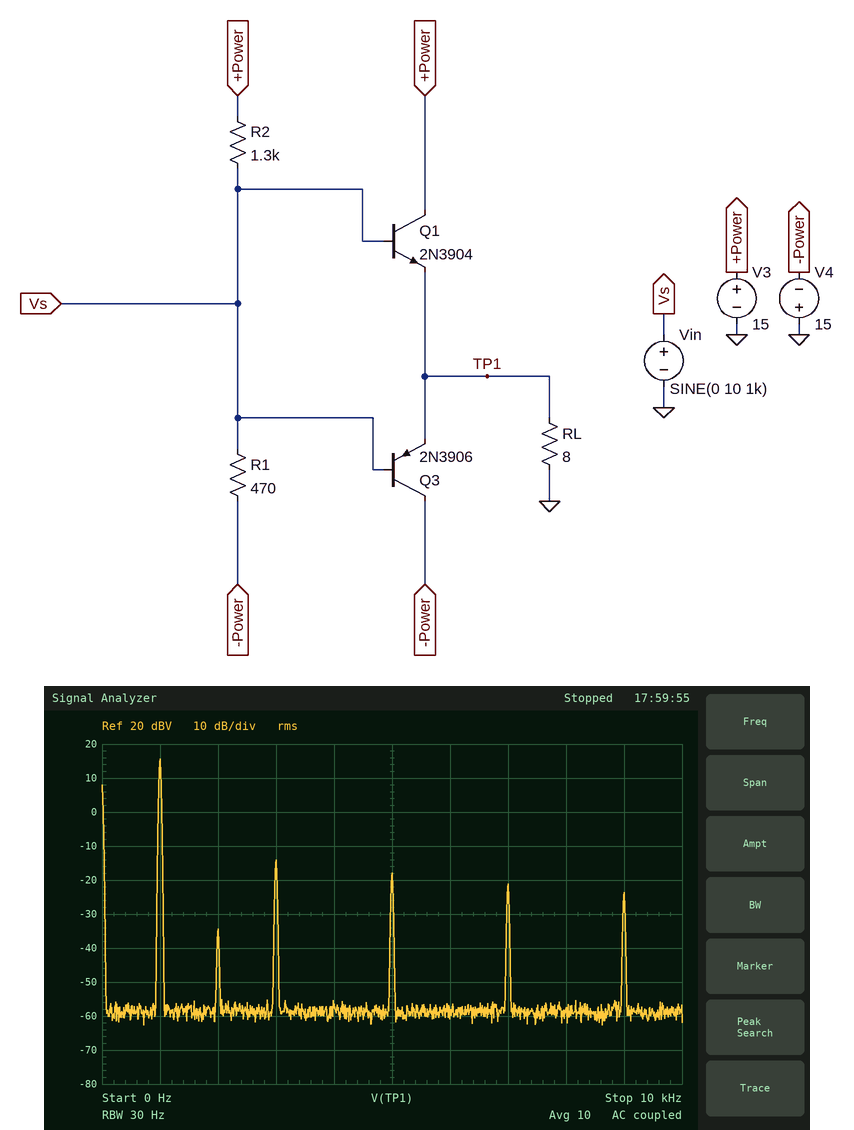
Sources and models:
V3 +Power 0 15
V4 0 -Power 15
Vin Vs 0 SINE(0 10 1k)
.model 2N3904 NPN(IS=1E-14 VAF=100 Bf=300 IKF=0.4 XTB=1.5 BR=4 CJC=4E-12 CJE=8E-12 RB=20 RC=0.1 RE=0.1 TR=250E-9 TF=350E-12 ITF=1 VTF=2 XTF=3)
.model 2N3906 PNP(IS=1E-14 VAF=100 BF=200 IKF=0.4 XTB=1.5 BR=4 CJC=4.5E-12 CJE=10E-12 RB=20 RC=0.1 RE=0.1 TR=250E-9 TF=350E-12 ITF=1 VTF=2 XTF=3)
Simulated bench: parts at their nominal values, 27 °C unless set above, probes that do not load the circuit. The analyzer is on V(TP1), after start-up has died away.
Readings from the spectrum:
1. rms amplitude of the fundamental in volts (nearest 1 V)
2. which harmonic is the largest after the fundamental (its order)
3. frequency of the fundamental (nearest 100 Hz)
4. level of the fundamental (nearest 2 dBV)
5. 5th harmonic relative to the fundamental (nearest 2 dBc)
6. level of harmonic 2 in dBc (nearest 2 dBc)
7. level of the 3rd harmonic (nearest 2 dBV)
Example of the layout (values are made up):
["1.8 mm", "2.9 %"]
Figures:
["6 V", "3", "1.0 kHz", "16 dBV", "-34 dBc", "-50 dBc", "-14 dBV"]
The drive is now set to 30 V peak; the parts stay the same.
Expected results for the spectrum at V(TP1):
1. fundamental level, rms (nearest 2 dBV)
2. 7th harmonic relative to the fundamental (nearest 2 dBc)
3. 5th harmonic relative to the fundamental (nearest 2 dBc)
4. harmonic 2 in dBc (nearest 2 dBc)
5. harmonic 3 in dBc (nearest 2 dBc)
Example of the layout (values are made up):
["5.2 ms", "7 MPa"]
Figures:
["22 dBV", "-30 dBc", "-34 dBc", "-58 dBc", "-14 dBc"]
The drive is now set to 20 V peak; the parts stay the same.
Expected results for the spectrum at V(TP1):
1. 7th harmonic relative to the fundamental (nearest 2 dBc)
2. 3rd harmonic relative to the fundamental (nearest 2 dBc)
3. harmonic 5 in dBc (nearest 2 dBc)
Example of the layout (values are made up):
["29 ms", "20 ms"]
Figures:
["-48 dBc", "-24 dBc", "-28 dBc"]
